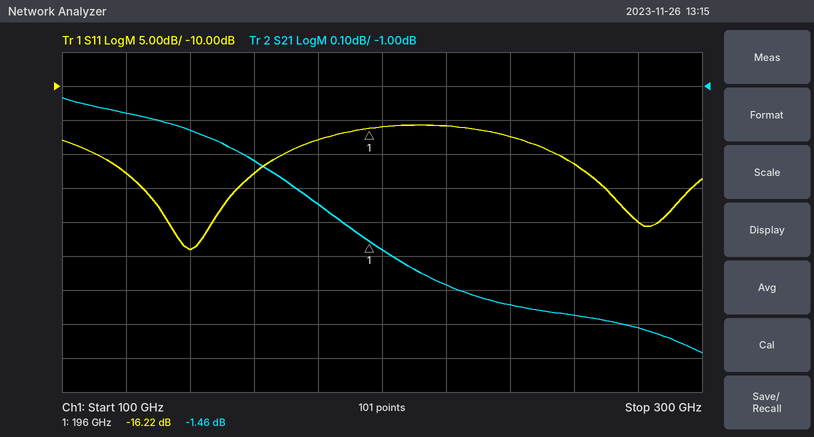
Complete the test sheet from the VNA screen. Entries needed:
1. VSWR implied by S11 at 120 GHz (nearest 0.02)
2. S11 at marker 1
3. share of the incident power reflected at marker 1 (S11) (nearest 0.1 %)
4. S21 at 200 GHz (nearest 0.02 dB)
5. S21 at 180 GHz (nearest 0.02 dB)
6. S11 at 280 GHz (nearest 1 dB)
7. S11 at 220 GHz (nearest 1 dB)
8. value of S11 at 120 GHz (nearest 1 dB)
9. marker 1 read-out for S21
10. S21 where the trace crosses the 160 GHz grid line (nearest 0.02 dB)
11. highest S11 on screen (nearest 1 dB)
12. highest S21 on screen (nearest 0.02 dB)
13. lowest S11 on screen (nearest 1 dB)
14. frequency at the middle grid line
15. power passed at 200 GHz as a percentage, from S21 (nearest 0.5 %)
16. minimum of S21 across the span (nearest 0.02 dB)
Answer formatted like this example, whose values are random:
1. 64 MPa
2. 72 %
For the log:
1. 1.16
2. -16.22 dB
3. 2.4 %
4. -1.48 dB
5. -1.34 dB
6. -30 dB
7. -16 dB
8. -23 dB
9. -1.46 dB
10. -1.22 dB
11. -16 dB
12. -1.04 dB
13. -34 dB
14. 200 GHz
15. 71.0 %
16. -1.78 dB
